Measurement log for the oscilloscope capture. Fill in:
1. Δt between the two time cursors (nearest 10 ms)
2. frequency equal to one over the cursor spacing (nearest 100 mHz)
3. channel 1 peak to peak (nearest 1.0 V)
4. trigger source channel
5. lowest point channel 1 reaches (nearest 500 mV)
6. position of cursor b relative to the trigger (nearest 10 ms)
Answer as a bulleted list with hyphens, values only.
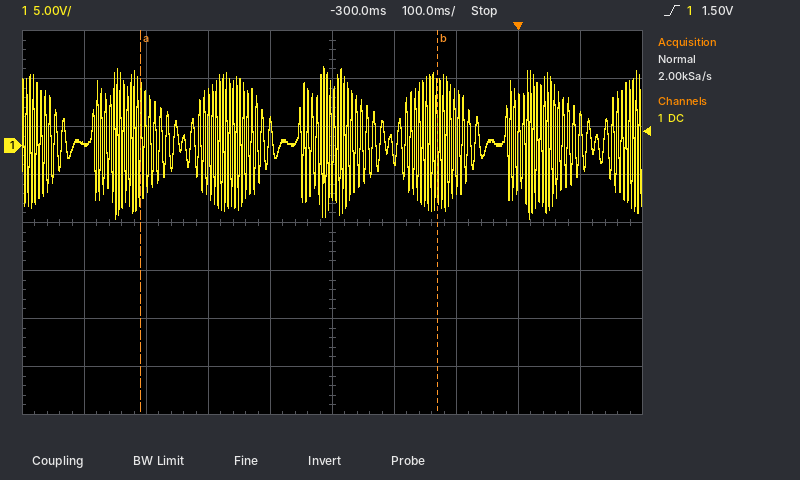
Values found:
- 480 ms
- 2.1 Hz
- 16.0 V
- channel 1
- -7.5 V
- -130 ms
